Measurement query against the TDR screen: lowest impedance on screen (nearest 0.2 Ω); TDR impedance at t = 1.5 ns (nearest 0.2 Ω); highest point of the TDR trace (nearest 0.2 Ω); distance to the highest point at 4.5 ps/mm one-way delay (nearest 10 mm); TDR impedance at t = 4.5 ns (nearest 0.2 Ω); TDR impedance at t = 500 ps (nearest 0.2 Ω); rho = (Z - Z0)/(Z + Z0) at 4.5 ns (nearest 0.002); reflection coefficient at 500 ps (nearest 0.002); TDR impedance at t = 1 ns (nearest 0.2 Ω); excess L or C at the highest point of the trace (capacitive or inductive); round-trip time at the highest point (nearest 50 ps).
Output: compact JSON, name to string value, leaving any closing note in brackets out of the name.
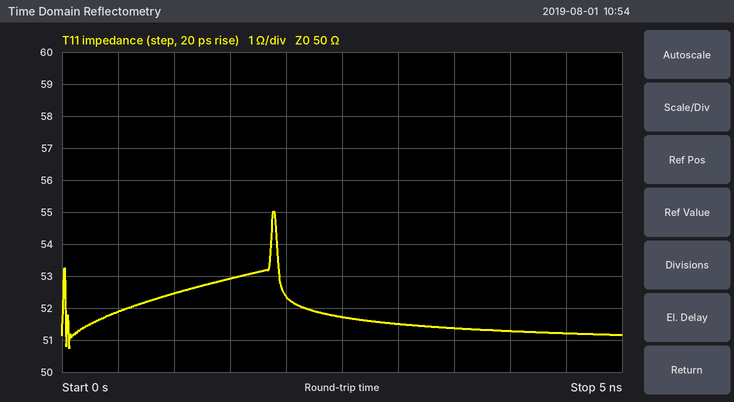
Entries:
{"lowest impedance on screen": "50.8 Ω", "TDR impedance at t = 1.5 ns": "53.0 Ω", "highest point of the TDR trace": "55.0 Ω", "distance to the highest point at 4.5 ps/mm one-way delay": "210 mm", "TDR impedance at t = 4.5 ns": "51.2 Ω", "TDR impedance at t = 500 ps": "51.8 Ω", "rho = (Z - Z0)/(Z + Z0) at 4.5 ns": "+0.012", "reflection coefficient at 500 ps": "+0.018", "TDR impedance at t = 1 ns": "52.4 Ω", "excess L or C at the highest point of the trace": "inductive", "round-trip time at the highest point": "1.90 ns"}
